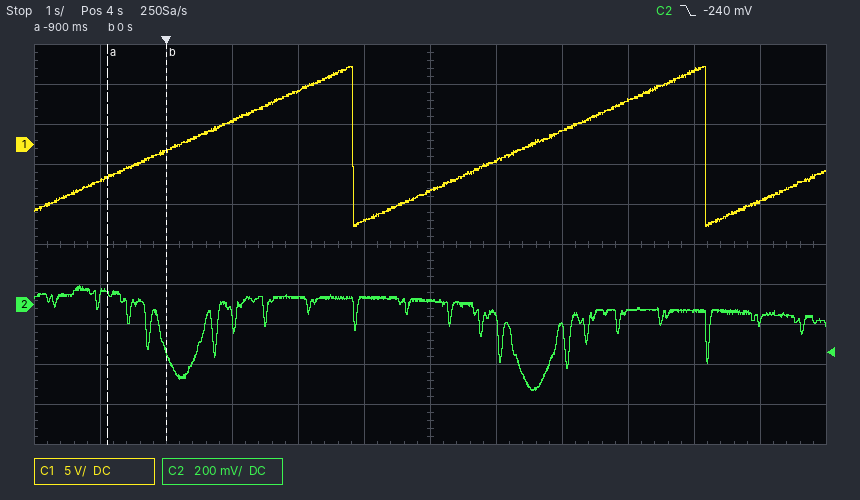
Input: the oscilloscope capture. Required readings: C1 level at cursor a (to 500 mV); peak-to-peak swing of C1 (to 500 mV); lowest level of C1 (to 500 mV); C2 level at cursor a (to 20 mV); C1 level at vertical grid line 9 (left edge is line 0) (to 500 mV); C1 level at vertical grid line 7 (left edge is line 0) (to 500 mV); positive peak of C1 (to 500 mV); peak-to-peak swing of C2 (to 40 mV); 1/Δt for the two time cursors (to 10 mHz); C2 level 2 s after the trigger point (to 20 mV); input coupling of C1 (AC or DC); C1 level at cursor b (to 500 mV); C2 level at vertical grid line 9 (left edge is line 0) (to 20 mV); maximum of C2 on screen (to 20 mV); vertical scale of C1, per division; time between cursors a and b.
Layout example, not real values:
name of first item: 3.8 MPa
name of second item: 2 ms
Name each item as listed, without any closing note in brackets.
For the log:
C1 level at cursor a: -4.0 V
peak-to-peak swing of C1: 20.0 V
lowest level of C1: -10.0 V
C2 level at cursor a: 60 mV
C1 level at vertical grid line 9 (left edge is line 0): 5.5 V
C1 level at vertical grid line 7 (left edge is line 0): -2.0 V
positive peak of C1: 10.0 V
peak-to-peak swing of C2: 520 mV
1/Δt for the two time cursors: 1.11 Hz
C2 level 2 s after the trigger point: 40 mV
input coupling of C1: DC
C1 level at cursor b: -1.0 V
C2 level at vertical grid line 9 (left edge is line 0): -40 mV
maximum of C2 on screen: 100 mV
vertical scale of C1, per division: 5 V
time between cursors a and b: 900 ms
